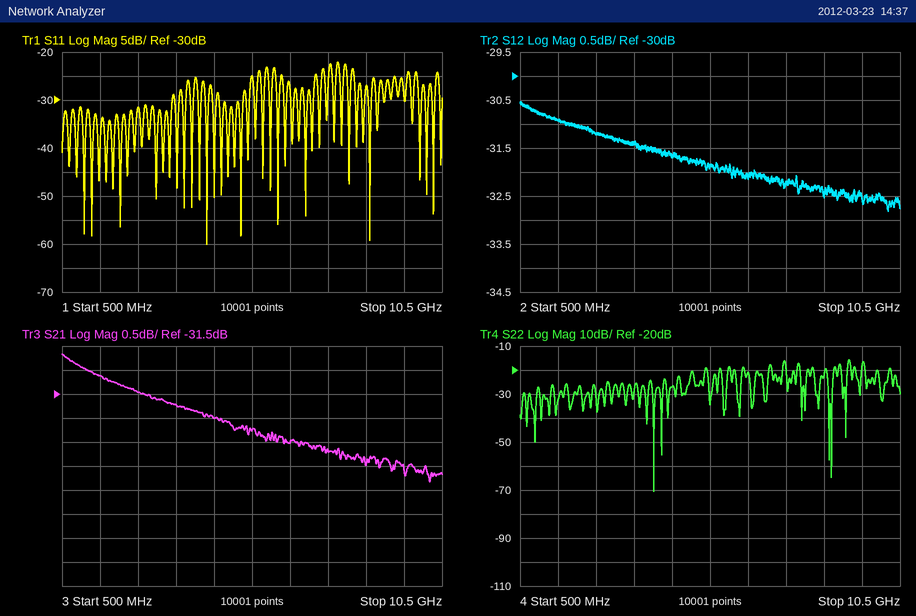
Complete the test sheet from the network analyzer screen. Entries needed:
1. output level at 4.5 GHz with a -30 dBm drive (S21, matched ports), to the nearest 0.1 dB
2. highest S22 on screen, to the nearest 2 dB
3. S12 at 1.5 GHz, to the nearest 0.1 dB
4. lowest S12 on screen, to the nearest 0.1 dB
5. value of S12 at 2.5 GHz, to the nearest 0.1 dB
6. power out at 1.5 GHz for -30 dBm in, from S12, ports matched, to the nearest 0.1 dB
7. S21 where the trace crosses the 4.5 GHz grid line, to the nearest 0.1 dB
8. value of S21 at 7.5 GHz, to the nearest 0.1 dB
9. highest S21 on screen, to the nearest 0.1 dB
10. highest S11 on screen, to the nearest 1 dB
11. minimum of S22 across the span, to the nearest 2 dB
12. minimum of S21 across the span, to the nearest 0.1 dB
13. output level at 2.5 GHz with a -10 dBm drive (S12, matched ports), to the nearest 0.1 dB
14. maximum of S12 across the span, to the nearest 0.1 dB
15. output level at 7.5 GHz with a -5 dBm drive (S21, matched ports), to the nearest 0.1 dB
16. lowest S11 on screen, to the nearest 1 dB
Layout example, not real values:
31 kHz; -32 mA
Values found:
-62.0 dBm; -16 dB; -30.9 dB; -32.8 dB; -31.2 dB; -60.9 dBm; -32.0 dB; -32.7 dB; -30.7 dB; -22 dB; -70 dB; -33.3 dB; -41.2 dBm; -30.5 dB; -37.7 dBm; -60 dB
